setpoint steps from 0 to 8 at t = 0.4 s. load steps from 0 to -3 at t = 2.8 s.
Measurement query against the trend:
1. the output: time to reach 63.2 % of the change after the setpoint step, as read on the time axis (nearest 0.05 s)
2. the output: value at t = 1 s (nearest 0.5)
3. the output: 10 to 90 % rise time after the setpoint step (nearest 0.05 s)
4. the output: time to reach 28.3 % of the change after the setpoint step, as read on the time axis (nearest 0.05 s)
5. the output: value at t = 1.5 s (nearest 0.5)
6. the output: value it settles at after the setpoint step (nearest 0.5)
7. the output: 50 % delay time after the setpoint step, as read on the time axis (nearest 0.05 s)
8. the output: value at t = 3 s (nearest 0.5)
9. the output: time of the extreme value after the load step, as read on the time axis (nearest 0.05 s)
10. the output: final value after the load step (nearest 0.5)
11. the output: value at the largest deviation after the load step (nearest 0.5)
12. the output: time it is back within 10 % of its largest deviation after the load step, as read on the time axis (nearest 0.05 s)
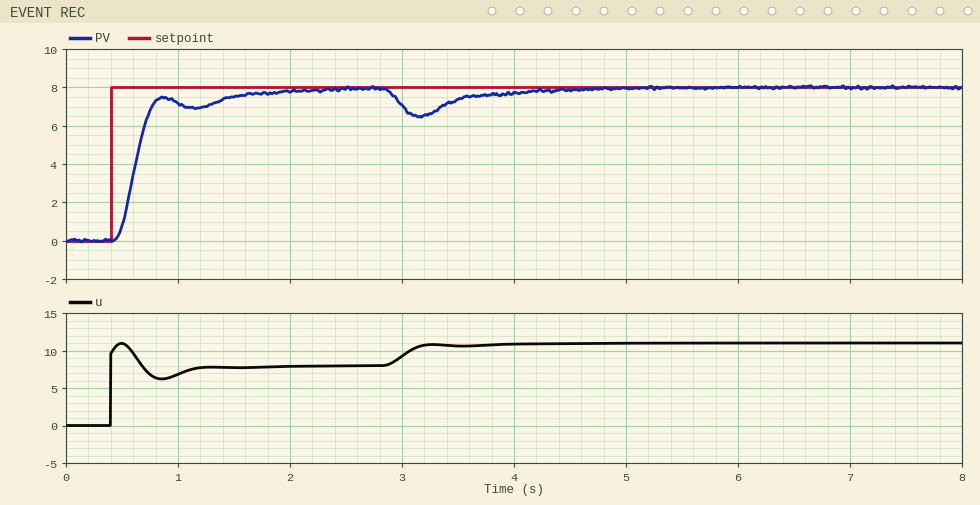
0.65 s
7.0
0.30 s
0.55 s
7.5
8.0
0.60 s
7.0
3.15 s
8.0
6.5
4.40 s
